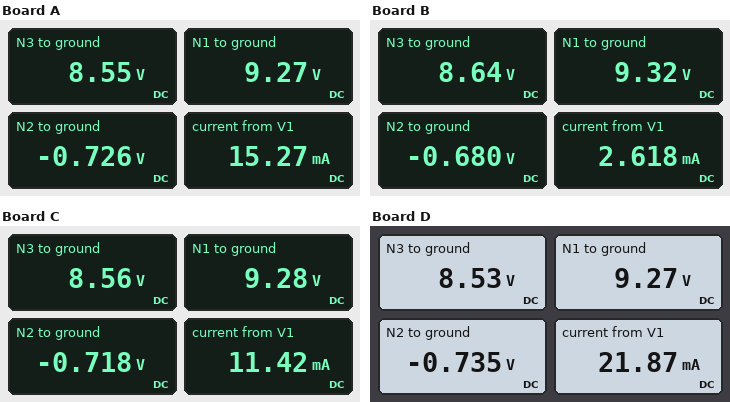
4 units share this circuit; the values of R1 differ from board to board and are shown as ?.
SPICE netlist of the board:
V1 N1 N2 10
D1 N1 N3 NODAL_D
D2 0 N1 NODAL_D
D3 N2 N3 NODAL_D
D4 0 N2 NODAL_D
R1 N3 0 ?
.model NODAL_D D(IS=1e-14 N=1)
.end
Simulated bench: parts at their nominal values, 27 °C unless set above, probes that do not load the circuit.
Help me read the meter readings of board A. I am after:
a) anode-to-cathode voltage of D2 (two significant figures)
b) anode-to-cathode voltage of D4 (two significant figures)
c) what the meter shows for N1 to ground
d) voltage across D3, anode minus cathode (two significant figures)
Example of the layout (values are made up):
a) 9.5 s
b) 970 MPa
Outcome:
a) -9.3 V
b) 730 mV
c) 9.27 V
d) -9.3 V
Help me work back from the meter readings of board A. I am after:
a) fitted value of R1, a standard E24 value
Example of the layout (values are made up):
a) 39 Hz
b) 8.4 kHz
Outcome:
a) 560 Ω
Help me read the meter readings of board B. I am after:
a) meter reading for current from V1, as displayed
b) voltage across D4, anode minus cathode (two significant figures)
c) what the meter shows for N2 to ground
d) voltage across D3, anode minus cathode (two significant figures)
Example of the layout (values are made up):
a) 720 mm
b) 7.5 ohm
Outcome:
a) 2.618 mA
b) 680 mV
c) -0.680 V
d) -9.3 V
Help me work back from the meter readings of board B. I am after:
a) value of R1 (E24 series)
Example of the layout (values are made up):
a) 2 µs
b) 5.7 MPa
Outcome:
a) 3.3 kΩ
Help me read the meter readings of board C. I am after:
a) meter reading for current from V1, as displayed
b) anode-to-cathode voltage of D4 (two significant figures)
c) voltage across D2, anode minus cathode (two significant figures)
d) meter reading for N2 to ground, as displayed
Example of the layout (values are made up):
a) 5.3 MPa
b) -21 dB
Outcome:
a) 11.42 mA
b) 720 mV
c) -9.3 V
d) -0.718 V
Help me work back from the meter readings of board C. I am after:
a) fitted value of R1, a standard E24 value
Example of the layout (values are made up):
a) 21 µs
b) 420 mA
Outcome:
a) 750 Ω
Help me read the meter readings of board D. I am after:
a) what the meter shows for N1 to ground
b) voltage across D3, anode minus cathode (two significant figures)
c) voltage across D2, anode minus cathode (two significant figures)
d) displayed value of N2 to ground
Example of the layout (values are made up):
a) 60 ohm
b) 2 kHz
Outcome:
a) 9.27 V
b) -9.3 V
c) -9.3 V
d) -0.735 V
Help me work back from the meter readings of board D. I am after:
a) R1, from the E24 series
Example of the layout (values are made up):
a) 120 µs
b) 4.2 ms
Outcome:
a) 390 Ω
